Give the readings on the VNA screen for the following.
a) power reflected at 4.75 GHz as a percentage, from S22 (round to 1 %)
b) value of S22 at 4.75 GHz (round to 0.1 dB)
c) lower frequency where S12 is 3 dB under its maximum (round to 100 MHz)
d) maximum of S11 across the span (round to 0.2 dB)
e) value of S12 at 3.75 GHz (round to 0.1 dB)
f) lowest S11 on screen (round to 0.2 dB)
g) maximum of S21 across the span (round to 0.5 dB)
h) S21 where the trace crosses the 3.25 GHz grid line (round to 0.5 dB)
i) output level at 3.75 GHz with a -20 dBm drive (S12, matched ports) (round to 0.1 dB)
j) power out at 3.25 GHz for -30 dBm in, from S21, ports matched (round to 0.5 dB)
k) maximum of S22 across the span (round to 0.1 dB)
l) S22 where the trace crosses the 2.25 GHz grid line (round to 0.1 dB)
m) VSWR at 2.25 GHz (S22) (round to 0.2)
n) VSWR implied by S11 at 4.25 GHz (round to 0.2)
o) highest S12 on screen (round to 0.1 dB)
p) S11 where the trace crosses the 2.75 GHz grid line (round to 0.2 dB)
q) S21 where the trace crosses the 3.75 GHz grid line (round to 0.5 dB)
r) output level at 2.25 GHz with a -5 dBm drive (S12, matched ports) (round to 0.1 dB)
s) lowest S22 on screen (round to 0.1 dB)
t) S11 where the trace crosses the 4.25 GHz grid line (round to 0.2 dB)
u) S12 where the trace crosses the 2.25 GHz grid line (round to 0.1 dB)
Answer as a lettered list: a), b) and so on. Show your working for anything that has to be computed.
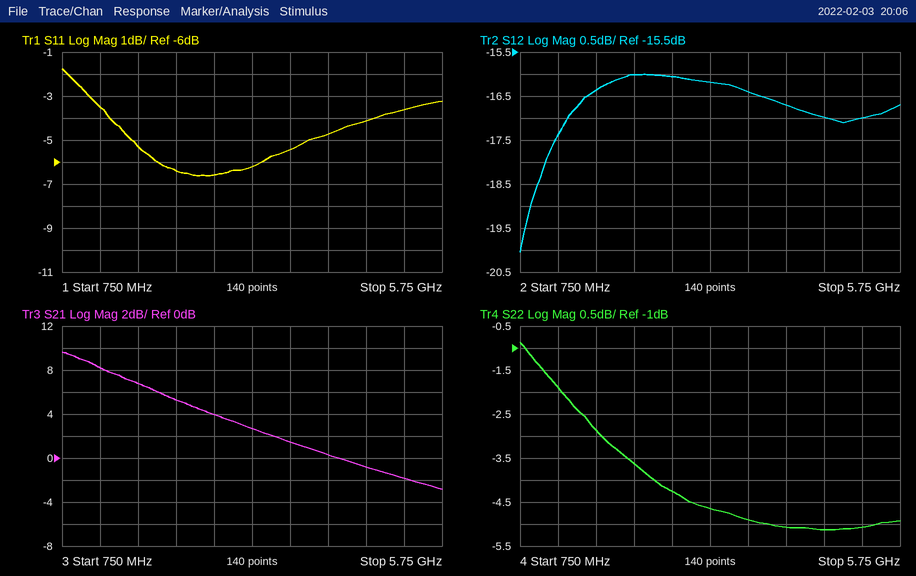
a) 10^(-5.1/10) ≈ 31 %
b) -5.1 dB
c) 900 MHz
d) -1.8 dB
e) -16.4 dB
f) -6.6 dB
g) 9.5 dB
h) 2.5 dB
i) -20 dBm + (-16.4 dB) = -36.4 dBm
j) -30 dBm + (2.5 dB) = -27.5 dBm
k) -0.9 dB
l) -3.6 dB
m) |Γ| = 10^(-3.6/20) = 0.6607; VSWR = (1 + 0.6607)/(1 − 0.6607) ≈ 4.89, so 4.8 to the nearest 0.2
n) |Γ| = 10^(-4.8/20) = 0.5754; VSWR = (1 + 0.5754)/(1 − 0.5754) ≈ 3.71, so 3.8 to the nearest 0.2
o) -16.0 dB
p) -6.6 dB
q) 1.5 dB
r) -5 dBm + (-16.0 dB) = -21.0 dBm
s) -5.1 dB
t) -4.8 dB
u) -16.0 dB
